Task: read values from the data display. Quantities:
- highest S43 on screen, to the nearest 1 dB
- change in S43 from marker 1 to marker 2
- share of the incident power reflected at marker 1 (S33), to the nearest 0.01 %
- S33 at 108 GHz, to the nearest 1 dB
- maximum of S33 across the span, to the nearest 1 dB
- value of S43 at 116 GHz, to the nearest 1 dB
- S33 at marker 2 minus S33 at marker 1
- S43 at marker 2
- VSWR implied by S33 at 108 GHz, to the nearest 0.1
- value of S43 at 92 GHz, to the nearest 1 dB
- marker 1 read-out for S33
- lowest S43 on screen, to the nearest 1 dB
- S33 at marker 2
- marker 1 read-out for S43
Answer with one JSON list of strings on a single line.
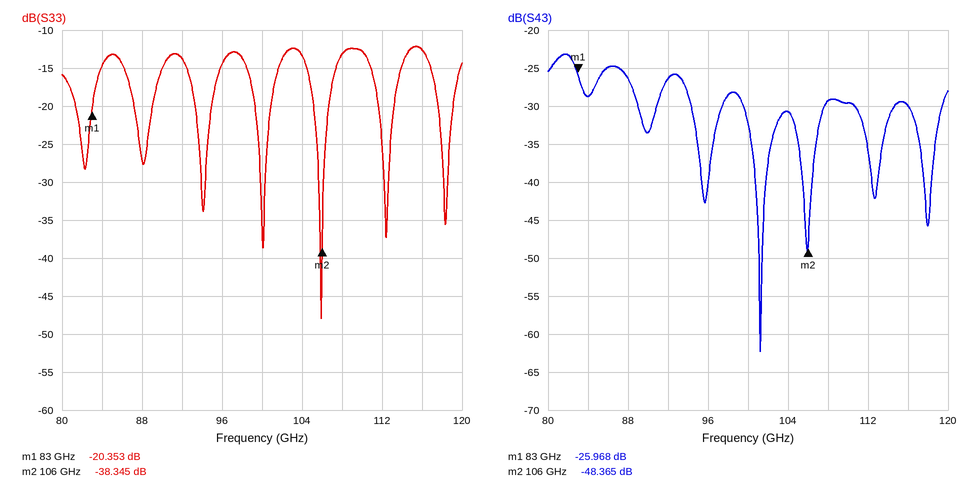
["-23 dB", "-22.397 dB", "0.92 %", "-13 dB", "-12 dB", "-30 dB", "-17.992 dB", "-48.365 dB", "1.6", "-26 dB", "-20.353 dB", "-62 dB", "-38.345 dB", "-25.968 dB"]
